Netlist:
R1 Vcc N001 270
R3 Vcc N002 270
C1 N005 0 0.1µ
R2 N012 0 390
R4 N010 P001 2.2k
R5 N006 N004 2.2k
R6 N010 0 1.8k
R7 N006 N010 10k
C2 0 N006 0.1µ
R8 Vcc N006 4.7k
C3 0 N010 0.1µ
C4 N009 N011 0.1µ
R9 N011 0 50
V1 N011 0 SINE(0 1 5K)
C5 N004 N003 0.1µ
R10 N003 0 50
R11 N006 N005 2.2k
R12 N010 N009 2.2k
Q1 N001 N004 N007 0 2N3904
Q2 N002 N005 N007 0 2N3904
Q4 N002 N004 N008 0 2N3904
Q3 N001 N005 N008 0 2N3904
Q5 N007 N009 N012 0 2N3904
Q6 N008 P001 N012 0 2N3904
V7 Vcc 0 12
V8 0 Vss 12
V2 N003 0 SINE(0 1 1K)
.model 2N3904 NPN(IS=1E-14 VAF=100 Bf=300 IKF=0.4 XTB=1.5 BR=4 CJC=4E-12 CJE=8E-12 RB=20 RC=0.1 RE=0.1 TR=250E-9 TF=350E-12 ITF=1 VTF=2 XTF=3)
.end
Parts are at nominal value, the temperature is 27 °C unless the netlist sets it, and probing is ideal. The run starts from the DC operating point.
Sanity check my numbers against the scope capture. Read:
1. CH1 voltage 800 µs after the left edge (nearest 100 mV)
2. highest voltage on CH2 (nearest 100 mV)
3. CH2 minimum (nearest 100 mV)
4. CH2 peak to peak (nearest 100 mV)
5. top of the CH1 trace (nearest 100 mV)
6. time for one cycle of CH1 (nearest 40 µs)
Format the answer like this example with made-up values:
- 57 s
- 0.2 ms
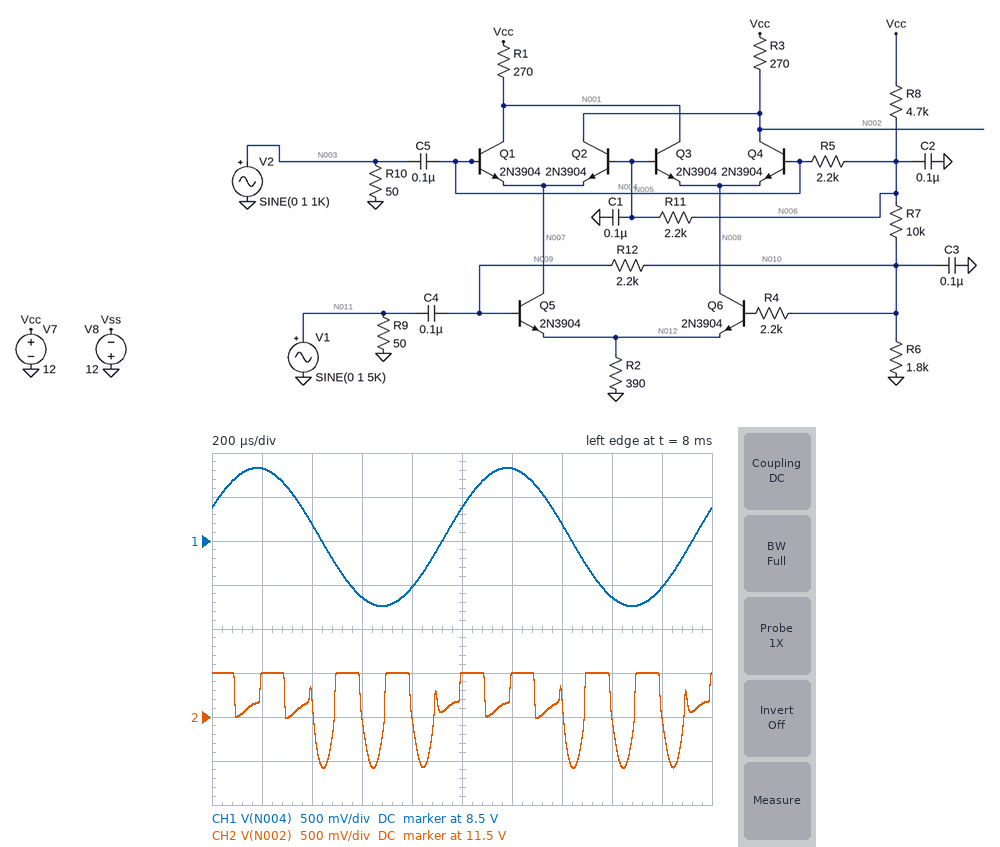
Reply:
- 8.0 V
- 12.0 V
- 10.9 V
- 1.1 V
- 9.3 V
- 1.00 ms
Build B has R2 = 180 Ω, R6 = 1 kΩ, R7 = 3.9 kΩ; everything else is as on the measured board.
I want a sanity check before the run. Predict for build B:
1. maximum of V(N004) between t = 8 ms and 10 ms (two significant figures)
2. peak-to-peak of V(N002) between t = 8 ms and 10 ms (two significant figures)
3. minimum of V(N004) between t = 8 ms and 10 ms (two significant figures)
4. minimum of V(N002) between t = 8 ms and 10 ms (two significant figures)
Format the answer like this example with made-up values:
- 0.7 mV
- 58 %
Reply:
- 6.9 V
- 2.2 V
- 5.3 V
- 9.8 V
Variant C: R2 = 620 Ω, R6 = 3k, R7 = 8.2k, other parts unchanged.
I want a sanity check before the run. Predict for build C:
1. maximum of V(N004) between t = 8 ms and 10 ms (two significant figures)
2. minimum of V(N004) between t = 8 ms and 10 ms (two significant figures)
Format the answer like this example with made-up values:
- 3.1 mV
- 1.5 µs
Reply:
- 9.2 V
- 7.6 V
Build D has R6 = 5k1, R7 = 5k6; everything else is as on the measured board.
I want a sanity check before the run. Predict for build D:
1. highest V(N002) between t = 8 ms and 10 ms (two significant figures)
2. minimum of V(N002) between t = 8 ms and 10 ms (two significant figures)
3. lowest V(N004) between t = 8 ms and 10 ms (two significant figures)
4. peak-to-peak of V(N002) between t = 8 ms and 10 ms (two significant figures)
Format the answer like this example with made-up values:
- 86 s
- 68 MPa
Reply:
- 12 V
- 9.2 V
- 7.4 V
- 2.8 V
